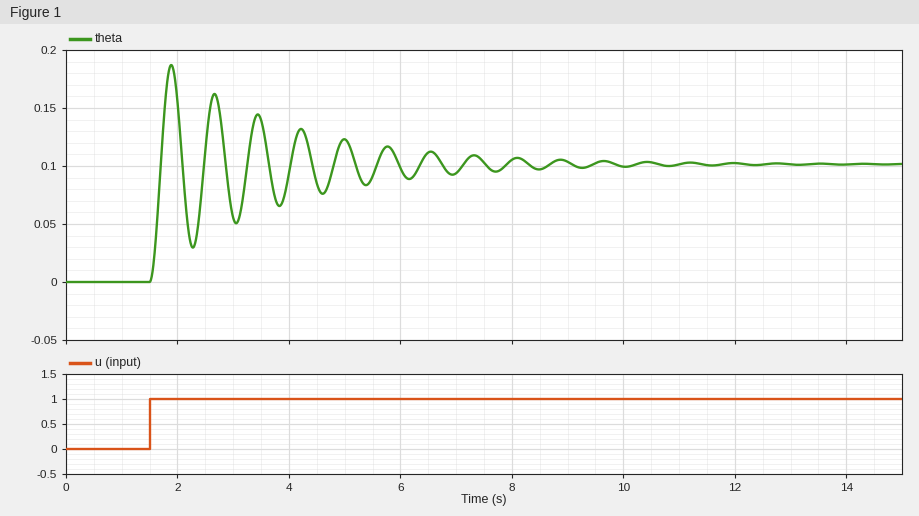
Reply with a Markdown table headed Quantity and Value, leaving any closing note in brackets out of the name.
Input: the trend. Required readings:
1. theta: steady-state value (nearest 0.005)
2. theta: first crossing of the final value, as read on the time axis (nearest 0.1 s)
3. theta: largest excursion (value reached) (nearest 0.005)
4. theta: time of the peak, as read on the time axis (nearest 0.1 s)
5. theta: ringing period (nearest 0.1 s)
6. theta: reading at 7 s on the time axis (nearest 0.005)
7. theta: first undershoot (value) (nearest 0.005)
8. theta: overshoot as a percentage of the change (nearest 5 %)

| Quantity | Value |
|---|---|
| theta: steady-state value | 0.100 |
| theta: first crossing of the final value, as read on the time axis | 1.7 s |
| theta: largest excursion (value reached) | 0.185 |
| theta: time of the peak, as read on the time axis | 1.9 s |
| theta: ringing period | 0.8 s |
| theta: reading at 7 s on the time axis | 0.095 |
| theta: first undershoot (value) | 0.030 |
| theta: overshoot as a percentage of the change | 85 % |
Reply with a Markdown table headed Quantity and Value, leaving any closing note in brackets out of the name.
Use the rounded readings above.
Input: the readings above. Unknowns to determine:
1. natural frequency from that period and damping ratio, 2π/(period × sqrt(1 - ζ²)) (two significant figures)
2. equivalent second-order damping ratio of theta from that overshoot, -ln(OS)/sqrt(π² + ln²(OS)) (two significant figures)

| Quantity | Value |
|---|---|
| natural frequency from that period and damping ratio, 2π/(period × sqrt(1 - ζ²)) | 7.9 rad/s |
| equivalent second-order damping ratio of theta from that overshoot, -ln(OS)/sqrt(π² + ln²(OS)) | 0.052 |
